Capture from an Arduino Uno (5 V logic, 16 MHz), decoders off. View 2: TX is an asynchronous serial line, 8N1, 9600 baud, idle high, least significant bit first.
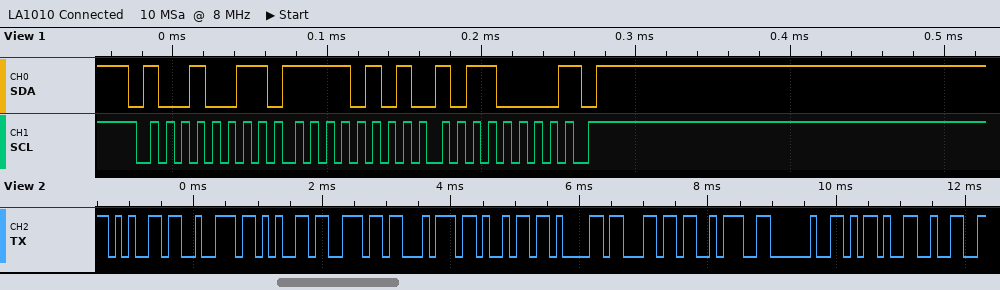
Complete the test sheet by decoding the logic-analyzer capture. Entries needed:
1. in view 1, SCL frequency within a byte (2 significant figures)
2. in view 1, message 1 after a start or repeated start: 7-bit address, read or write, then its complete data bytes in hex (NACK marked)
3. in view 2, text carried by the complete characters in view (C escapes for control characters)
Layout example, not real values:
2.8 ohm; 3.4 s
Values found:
100 kHz; 0x49 read: F5 B0 NACK; "erential: -2"
